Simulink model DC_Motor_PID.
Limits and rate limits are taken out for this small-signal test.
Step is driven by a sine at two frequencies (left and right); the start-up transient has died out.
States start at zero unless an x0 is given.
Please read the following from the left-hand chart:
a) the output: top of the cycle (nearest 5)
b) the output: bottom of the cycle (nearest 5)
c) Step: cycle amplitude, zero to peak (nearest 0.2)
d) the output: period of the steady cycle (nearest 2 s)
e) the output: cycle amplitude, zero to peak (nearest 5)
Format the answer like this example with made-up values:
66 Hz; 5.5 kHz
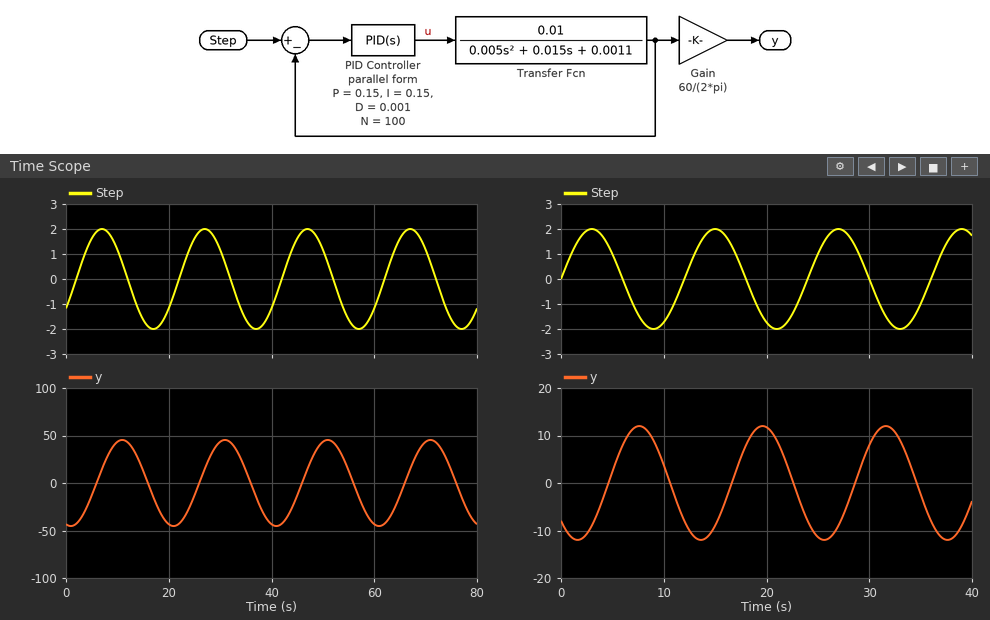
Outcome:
45; -45; 2.0; 20 s; 45
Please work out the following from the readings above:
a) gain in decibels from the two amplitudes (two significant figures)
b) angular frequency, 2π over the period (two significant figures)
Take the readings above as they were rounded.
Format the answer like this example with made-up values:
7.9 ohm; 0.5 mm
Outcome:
27 dB; 0.31 rad/s
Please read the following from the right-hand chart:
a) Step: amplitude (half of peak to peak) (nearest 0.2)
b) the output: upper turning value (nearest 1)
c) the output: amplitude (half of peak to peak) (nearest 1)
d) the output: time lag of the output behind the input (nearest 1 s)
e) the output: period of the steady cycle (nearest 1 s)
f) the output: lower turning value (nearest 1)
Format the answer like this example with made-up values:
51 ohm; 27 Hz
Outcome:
2.0; 12; 12; 5 s; 12 s; -12
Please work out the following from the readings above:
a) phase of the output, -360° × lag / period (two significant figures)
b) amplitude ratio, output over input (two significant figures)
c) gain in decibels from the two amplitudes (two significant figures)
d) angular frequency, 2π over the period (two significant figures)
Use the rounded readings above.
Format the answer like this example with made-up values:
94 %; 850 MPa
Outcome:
-150°; 6.0; 16 dB; 0.52 rad/s
